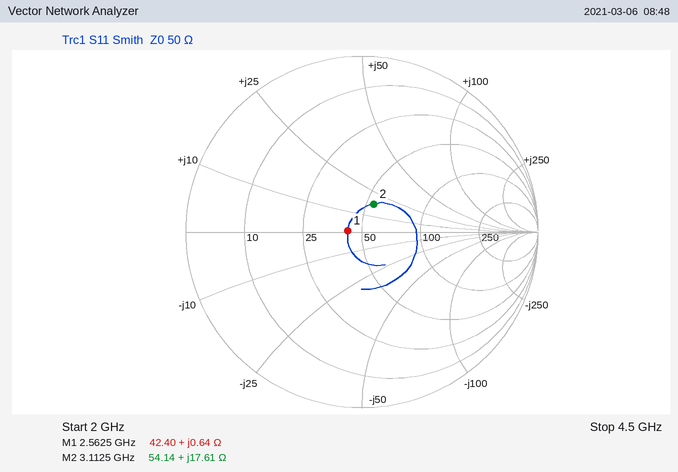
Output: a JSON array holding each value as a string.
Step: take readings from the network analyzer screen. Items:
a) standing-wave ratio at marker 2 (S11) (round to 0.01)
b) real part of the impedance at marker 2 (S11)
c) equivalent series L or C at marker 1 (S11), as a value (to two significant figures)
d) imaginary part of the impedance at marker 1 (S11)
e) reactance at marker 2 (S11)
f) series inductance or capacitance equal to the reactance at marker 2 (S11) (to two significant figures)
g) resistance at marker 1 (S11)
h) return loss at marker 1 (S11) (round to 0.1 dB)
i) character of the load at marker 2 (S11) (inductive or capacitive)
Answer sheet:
["1.41", "54.14 Ω", "40 pH", "+0.64 Ω", "+17.61 Ω", "900 pH", "42.40 Ω", "21.7 dB", "inductive"]
